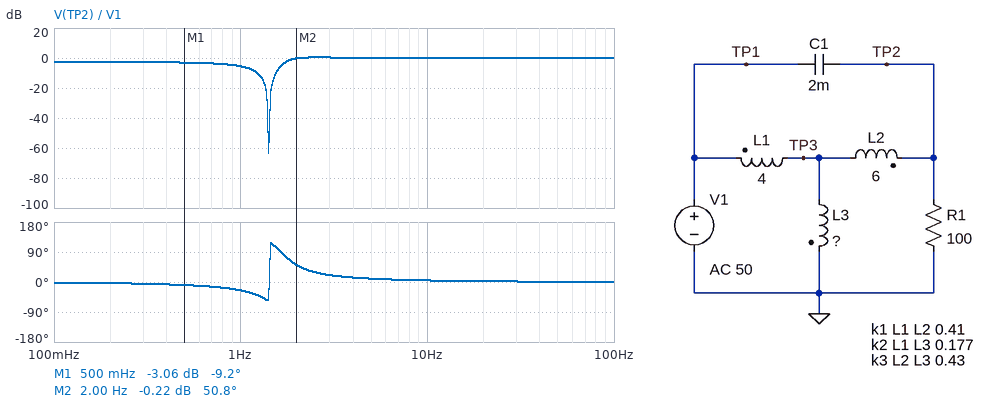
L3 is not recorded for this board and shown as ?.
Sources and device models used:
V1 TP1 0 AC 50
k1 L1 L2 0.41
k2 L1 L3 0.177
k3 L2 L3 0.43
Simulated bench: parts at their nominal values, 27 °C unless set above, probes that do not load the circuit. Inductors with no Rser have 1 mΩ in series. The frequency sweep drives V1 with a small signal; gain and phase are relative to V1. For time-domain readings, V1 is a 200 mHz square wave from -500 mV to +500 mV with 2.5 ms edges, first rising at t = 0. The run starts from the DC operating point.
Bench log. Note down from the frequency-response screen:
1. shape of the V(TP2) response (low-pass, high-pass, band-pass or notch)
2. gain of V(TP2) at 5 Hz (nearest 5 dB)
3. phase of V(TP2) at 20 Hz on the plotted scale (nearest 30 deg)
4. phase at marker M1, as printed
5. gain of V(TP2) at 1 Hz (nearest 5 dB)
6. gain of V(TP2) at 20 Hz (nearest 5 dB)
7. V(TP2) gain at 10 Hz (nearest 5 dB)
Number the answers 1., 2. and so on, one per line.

1. notch
2. 0 dB
3. 0 deg
4. -9.2 deg
5. -5 dB
6. 0 dB
7. 0 dB
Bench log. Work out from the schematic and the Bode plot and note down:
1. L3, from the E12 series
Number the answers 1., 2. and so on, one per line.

1. 18 H
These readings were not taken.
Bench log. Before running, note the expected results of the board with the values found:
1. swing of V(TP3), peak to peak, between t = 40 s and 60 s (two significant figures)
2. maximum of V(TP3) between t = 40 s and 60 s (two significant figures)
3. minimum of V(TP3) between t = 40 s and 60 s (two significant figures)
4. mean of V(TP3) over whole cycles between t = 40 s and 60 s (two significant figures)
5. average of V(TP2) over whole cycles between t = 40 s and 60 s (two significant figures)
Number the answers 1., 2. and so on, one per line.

1. 1.0 V
2. 690 mV
3. -320 mV
4. 180 mV
5. 120 mV
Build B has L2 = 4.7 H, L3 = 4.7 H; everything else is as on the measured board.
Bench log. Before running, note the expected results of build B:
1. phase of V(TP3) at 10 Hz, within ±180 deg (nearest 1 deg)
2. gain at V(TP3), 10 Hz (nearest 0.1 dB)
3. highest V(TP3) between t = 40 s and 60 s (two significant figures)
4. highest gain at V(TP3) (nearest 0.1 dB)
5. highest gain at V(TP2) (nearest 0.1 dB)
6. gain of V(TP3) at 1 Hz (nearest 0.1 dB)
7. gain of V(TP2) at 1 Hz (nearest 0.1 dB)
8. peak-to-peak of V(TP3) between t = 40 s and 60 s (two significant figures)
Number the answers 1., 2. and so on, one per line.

1. 1 deg
2. -3.8 dB
3. 390 mV
4. -3.5 dB
5. 2.9 dB
6. -5.9 dB
7. -9.9 dB
8. 730 mV
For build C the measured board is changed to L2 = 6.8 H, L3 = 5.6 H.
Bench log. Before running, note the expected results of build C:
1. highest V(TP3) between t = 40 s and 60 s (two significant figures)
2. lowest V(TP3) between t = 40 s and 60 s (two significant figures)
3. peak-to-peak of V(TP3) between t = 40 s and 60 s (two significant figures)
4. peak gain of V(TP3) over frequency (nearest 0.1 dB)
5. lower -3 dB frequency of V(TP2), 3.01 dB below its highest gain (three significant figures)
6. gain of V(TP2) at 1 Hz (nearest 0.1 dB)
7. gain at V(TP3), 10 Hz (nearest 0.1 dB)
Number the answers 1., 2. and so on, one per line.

1. 390 mV
2. -290 mV
3. 680 mV
4. -3.8 dB
5. 1.59 Hz
6. -12.9 dB
7. -3.9 dB
